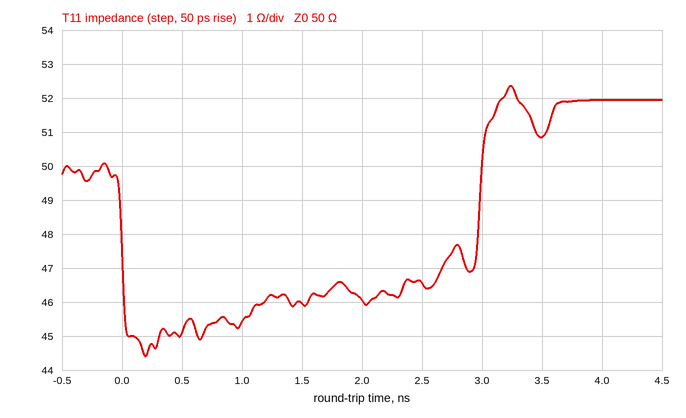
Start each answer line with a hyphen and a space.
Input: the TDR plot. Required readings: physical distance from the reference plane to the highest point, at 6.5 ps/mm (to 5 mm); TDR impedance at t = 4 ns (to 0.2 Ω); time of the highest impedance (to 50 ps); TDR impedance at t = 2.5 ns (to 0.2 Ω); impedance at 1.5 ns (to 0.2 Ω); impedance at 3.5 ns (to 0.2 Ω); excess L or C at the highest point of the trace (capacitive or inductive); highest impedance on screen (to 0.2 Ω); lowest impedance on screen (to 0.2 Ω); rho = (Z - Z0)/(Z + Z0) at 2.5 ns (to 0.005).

- 250 mm
- 52.0 Ω
- 3.25 ns
- 46.6 Ω
- 46.0 Ω
- 50.8 Ω
- inductive
- 52.4 Ω
- 44.4 Ω
- -0.035
